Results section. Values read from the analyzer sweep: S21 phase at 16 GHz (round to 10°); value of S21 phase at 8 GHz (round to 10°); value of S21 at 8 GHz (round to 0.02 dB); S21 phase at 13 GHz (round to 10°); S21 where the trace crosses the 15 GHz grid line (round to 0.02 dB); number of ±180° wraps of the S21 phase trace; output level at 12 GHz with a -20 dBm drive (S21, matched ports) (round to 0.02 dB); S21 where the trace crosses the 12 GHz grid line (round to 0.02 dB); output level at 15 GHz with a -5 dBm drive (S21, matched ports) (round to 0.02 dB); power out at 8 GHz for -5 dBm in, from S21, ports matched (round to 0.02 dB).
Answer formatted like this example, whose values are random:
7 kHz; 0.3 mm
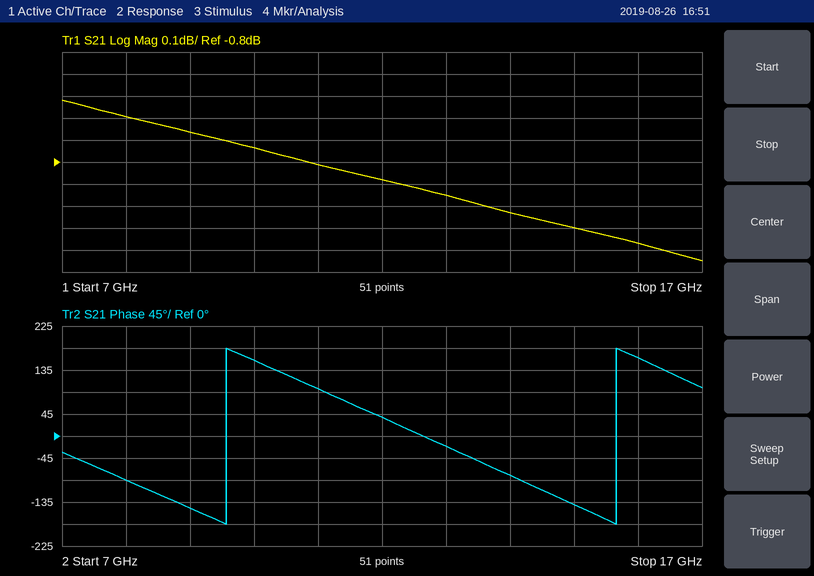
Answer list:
160°; -90°; -0.60 dB; -20°; -1.10 dB; 2; -20.88 dBm; -0.88 dB; -6.10 dBm; -5.60 dBm
